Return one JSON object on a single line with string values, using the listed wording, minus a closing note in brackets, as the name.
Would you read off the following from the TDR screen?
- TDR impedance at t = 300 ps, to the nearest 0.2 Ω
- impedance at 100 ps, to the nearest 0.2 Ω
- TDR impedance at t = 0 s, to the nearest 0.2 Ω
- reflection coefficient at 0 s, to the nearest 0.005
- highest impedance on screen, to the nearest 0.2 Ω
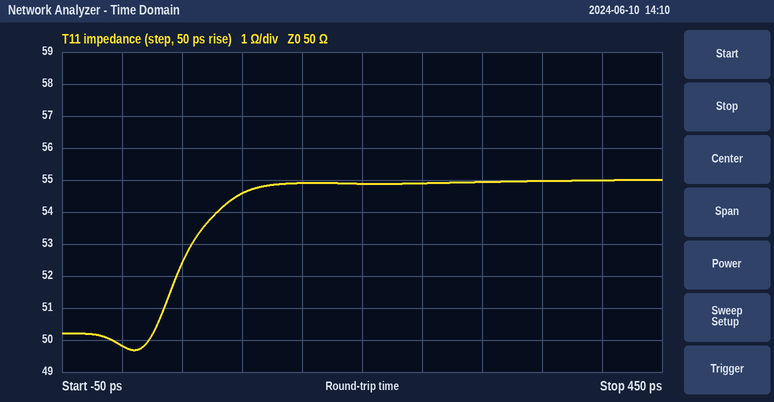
{"TDR impedance at t = 300 ps, to the nearest 0.2 Ω": "55.0 Ω", "impedance at 100 ps, to the nearest 0.2 Ω": "54.6 Ω", "TDR impedance at t = 0 s, to the nearest 0.2 Ω": "49.8 Ω", "reflection coefficient at 0 s, to the nearest 0.005": "0.000", "highest impedance on screen, to the nearest 0.2 Ω": "55.0 Ω"}
